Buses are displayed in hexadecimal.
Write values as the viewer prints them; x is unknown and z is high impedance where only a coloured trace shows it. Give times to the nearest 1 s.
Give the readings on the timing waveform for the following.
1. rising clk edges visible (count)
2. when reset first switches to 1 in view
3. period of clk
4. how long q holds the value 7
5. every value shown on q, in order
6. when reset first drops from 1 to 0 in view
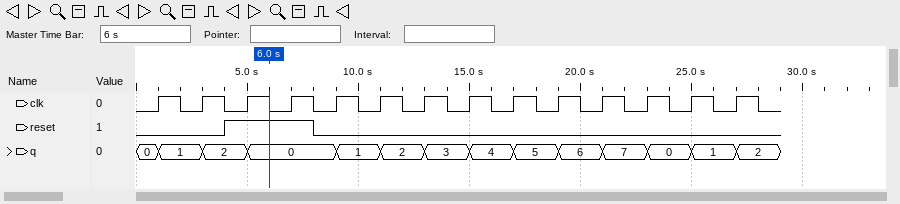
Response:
14
4 s
2 s
2 s
0, 1, 2, 0, 1, 2, 3, 4, 5, 6, 7, 0, 1, 2
8 s
